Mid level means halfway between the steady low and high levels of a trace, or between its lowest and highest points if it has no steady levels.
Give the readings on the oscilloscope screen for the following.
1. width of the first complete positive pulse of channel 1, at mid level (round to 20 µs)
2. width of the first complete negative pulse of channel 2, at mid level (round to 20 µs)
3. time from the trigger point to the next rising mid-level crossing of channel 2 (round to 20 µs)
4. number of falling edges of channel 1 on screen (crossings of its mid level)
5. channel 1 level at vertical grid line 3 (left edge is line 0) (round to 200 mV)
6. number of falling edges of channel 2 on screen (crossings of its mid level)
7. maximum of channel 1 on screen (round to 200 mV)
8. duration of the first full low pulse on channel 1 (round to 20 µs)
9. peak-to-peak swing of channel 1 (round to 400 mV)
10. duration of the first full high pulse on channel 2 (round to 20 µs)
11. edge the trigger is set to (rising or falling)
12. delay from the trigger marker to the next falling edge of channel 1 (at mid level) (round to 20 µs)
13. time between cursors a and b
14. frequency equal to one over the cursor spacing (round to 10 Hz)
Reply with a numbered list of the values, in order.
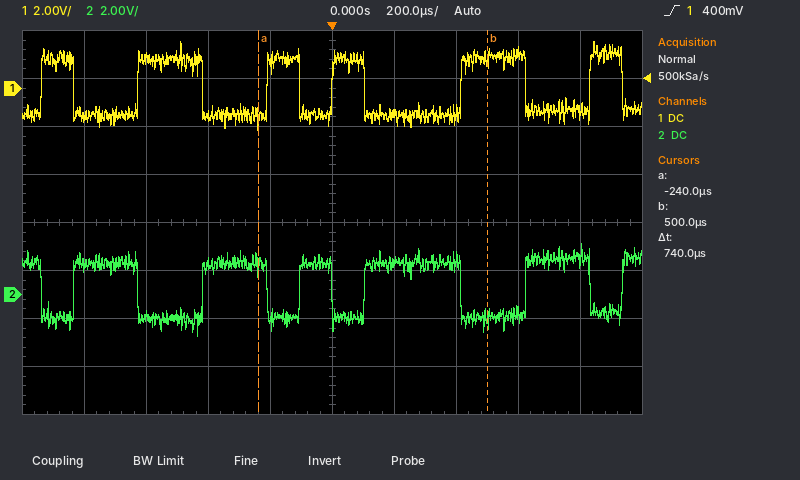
1. 100 µs
2. 100 µs
3. 100 µs
4. 6
5. -1.2 V
6. 6
7. 2.0 V
8. 200 µs
9. 3.6 V
10. 200 µs
11. rising
12. 100 µs
13. 740 µs
14. 1.35 kHz
